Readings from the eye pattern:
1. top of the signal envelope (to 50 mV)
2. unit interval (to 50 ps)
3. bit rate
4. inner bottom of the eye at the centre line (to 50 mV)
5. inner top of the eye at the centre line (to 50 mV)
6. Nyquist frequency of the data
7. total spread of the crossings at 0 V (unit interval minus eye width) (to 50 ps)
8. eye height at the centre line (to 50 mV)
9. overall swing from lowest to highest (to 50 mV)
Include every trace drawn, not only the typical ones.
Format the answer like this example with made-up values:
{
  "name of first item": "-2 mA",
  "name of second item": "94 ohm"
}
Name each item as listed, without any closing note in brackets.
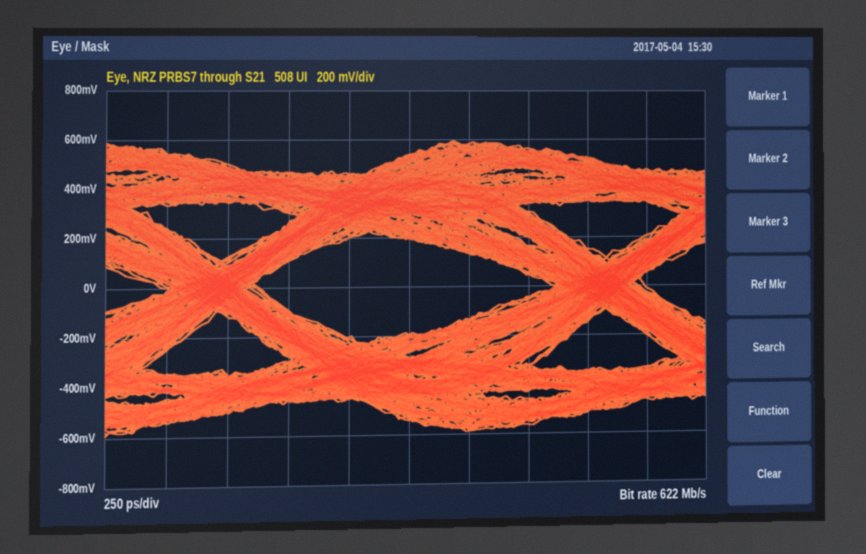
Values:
{
  "top of the signal envelope": "600 mV",
  "unit interval": "1.60 ns",
  "bit rate": "622 Mb/s",
  "inner bottom of the eye at the centre line": "-200 mV",
  "inner top of the eye at the centre line": "200 mV",
  "Nyquist frequency of the data": "311 MHz",
  "total spread of the crossings at 0 V (unit interval minus eye width)": "400 ps",
  "eye height at the centre line": "400 mV",
  "overall swing from lowest to highest": "1.20 V"
}
